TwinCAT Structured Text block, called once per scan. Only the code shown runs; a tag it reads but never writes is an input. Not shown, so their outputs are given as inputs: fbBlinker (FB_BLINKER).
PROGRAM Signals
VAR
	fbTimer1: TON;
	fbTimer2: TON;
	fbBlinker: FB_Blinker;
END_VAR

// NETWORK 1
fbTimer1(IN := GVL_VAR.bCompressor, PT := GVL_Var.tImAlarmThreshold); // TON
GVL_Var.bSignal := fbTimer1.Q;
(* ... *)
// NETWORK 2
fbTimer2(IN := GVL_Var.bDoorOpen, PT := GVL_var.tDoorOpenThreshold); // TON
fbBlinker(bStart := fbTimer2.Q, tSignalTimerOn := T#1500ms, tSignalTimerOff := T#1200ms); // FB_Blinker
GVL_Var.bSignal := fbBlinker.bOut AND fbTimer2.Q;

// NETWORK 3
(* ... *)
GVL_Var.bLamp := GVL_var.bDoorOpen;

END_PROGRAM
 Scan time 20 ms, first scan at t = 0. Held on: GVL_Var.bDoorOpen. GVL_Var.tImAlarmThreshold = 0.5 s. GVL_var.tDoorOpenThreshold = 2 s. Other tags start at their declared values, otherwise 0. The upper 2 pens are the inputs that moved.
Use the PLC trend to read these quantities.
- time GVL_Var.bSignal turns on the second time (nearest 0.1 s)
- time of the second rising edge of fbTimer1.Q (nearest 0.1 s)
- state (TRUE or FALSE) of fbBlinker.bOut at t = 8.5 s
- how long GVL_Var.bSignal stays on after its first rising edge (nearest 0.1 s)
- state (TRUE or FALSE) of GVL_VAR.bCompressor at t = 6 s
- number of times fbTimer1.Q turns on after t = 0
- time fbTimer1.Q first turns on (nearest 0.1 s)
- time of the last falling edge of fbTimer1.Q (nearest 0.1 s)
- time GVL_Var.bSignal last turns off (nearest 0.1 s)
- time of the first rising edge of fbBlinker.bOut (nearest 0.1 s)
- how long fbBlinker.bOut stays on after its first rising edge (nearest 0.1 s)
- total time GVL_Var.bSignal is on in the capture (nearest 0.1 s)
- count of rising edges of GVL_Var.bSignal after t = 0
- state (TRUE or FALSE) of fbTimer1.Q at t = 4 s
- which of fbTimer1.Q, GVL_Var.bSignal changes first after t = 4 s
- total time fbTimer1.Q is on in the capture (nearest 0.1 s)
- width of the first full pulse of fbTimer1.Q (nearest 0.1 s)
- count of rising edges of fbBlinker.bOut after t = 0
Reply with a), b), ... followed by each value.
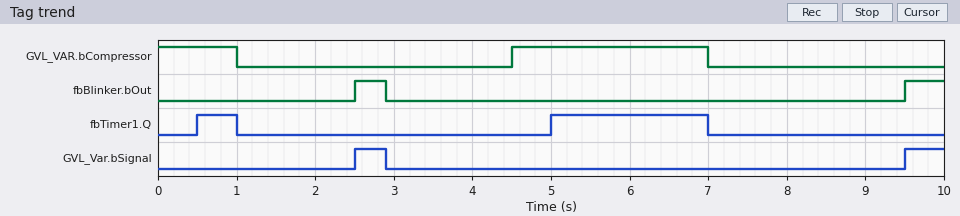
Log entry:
a) 9.5 s
b) 5.0 s
c) FALSE
d) 0.4 s
e) TRUE
f) 2
g) 0.5 s
h) 7.0 s
i) 2.9 s
j) 2.5 s
k) 0.4 s
l) 0.9 s
m) 2
n) FALSE
o) fbTimer1.Q
p) 2.5 s
q) 0.5 s
r) 2
